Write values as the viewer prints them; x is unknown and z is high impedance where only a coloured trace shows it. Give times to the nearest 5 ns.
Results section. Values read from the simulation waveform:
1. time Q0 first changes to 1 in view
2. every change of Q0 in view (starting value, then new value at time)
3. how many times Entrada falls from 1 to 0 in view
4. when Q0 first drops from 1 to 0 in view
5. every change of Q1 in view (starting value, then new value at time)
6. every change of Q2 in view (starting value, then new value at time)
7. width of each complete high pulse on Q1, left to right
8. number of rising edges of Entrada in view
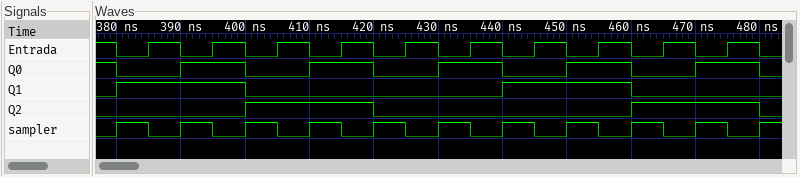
390 ns
1, 0 at 380 ns, 1 at 390 ns, 0 at 400 ns, 1 at 410 ns, 0 at 420 ns, 1 at 430 ns, 0 at 440 ns, 1 at 450 ns, 0 at 460 ns, 1 at 470 ns, 0 at 480 ns
11
380 ns
0, 1 at 380 ns, 0 at 400 ns, 1 at 440 ns, 0 at 460 ns
0, 1 at 400 ns, 0 at 420 ns, 1 at 460 ns, 0 at 480 ns
20 ns, 20 ns
10
